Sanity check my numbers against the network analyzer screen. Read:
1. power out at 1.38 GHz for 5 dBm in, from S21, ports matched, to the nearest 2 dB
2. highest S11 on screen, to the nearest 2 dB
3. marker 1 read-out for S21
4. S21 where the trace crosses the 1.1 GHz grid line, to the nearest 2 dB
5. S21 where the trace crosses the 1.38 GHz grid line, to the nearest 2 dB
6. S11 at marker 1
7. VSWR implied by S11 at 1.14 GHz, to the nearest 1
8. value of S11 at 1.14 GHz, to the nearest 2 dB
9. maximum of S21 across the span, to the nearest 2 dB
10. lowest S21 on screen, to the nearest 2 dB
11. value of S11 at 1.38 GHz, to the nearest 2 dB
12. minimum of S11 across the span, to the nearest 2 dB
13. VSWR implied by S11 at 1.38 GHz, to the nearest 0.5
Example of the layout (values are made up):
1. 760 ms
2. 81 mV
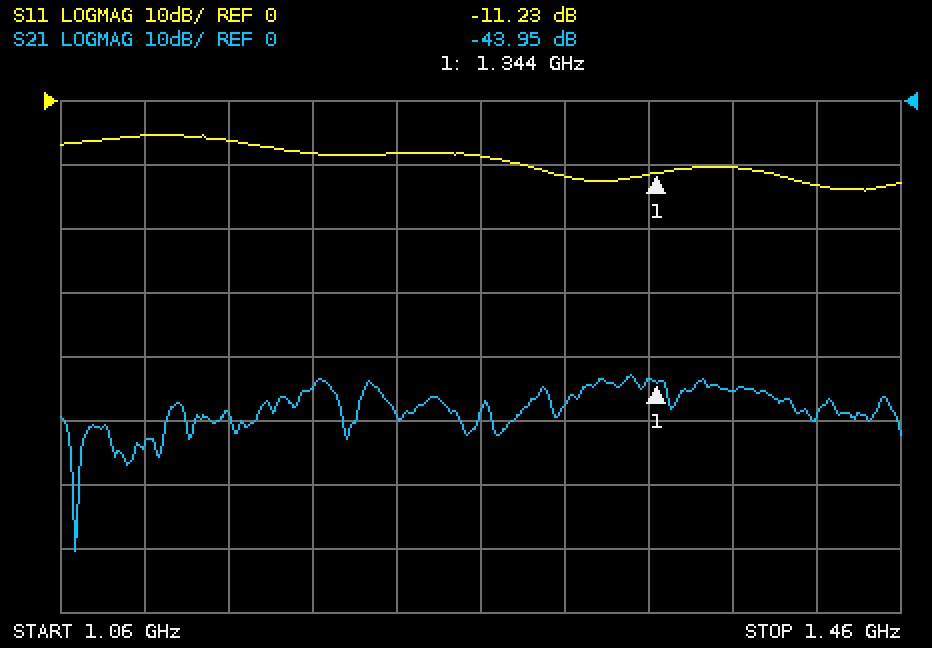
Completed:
1. -40 dBm
2. -6 dB
3. -43.95 dB
4. -54 dB
5. -46 dB
6. -11.23 dB
7. 3
8. -6 dB
9. -42 dB
10. -70 dB
11. -10 dB
12. -14 dB
13. 2.0
